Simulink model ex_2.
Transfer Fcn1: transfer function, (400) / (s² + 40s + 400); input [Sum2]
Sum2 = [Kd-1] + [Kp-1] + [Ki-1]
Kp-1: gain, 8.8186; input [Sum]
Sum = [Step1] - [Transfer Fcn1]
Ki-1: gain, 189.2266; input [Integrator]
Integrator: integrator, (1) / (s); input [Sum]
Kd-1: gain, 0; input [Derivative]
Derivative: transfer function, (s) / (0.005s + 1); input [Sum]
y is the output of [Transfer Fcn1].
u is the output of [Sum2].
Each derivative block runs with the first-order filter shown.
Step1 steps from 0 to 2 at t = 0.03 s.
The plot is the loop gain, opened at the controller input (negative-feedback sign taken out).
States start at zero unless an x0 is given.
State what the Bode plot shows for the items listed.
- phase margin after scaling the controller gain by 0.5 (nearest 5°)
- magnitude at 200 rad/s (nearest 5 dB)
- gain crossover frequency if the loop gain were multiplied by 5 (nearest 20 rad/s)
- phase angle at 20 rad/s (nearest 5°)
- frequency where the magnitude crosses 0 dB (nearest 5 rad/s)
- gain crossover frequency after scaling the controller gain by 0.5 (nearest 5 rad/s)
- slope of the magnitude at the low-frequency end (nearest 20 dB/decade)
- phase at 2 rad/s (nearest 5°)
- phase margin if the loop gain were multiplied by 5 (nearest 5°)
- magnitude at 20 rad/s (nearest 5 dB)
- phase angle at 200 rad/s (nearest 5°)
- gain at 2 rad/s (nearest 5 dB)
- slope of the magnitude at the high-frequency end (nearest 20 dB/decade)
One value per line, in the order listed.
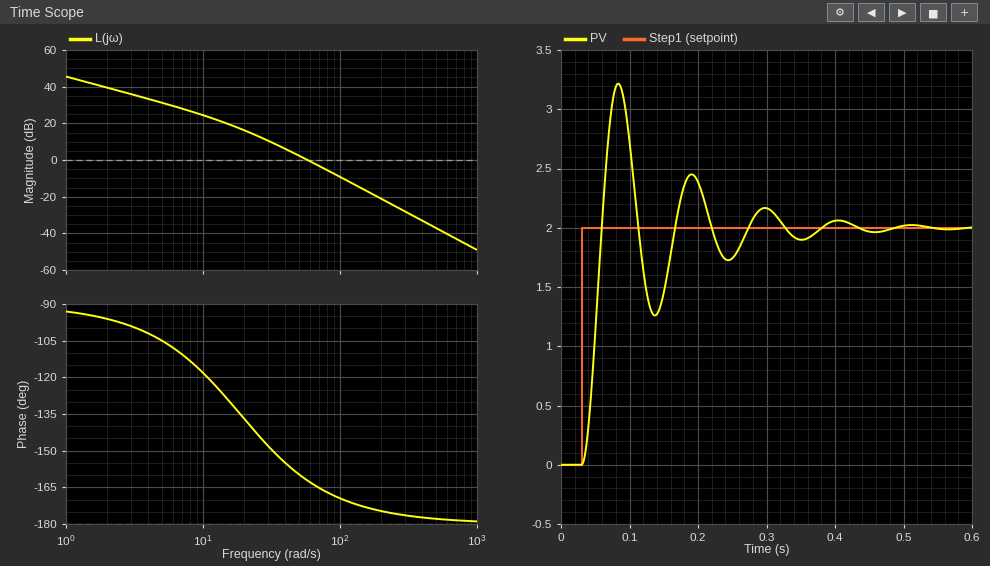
25°
-20 dB
140 rad/s
-135°
60 rad/s
40 rad/s
-20 dB/decade
-95°
10°
15 dB
-175°
40 dB
-40 dB/decade
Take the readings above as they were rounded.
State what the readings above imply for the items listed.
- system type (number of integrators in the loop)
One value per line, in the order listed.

1
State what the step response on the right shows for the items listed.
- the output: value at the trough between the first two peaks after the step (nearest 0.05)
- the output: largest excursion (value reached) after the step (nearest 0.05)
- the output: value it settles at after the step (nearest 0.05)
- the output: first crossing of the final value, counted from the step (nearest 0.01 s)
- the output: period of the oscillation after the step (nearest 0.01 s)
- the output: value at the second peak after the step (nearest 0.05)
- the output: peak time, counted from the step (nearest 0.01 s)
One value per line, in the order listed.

1.25
3.20
2.00
0.03 s
0.11 s
2.45
0.05 s
